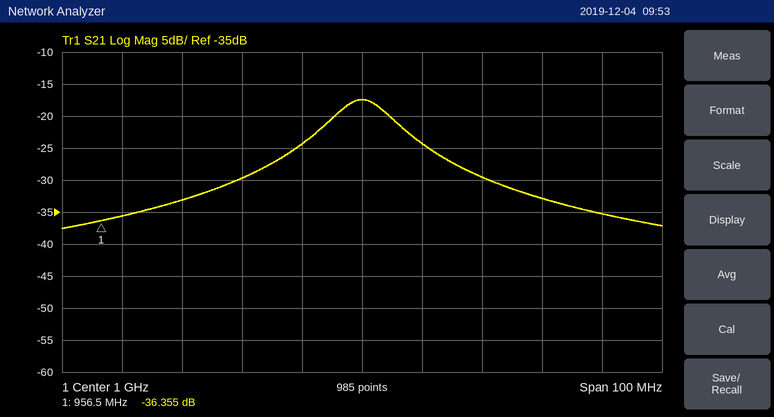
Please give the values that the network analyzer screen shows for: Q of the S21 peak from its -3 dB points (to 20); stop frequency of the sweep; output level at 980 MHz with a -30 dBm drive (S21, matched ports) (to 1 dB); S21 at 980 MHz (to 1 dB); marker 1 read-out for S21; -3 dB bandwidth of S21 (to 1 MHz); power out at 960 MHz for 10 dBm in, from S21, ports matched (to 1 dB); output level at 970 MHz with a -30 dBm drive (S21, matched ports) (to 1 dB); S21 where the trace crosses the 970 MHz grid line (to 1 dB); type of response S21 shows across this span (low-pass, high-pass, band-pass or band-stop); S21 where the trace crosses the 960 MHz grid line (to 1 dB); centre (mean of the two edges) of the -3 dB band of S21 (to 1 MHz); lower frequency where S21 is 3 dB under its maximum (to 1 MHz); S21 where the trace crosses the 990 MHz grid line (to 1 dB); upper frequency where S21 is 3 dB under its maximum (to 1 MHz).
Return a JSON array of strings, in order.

["100", "1.05 GHz", "-60 dBm", "-30 dB", "-36.355 dB", "10 MHz", "-26 dBm", "-63 dBm", "-33 dB", "band-pass", "-36 dB", "1.000 GHz", "995 MHz", "-24 dB", "1.005 GHz"]
